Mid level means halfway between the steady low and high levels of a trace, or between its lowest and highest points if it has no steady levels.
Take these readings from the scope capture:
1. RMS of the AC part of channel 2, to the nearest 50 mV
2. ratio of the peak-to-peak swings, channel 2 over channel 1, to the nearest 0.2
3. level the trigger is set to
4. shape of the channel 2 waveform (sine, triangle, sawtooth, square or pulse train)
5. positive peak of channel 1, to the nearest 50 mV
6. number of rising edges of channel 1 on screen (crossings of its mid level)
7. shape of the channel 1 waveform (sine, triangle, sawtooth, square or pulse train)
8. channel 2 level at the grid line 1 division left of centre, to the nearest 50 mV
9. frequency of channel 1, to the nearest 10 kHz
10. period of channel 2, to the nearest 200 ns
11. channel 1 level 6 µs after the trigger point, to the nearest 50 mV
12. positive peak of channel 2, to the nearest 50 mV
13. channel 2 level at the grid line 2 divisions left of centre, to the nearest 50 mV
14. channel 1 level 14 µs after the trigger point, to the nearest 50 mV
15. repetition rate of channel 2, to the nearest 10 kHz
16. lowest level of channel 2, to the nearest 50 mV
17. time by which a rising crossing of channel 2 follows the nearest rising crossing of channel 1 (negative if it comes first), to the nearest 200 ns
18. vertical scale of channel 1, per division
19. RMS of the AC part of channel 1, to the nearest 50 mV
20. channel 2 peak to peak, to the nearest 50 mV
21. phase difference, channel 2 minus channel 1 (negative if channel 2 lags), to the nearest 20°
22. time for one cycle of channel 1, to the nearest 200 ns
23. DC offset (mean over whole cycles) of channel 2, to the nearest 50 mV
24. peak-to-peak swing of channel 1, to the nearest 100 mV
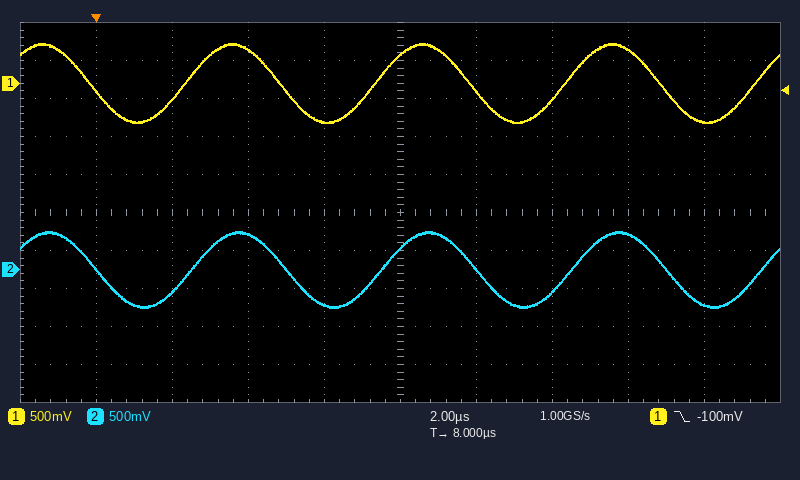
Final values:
350 mV
1.0
-100 mV
sine
500 mV
4
sine
-450 mV
200 kHz
5.0 µs
-500 mV
500 mV
450 mV
450 mV
200 kHz
-500 mV
+200 ns
500 mV
350 mV
1.00 V
-20°
5.0 µs
0 mV
1.00 V
